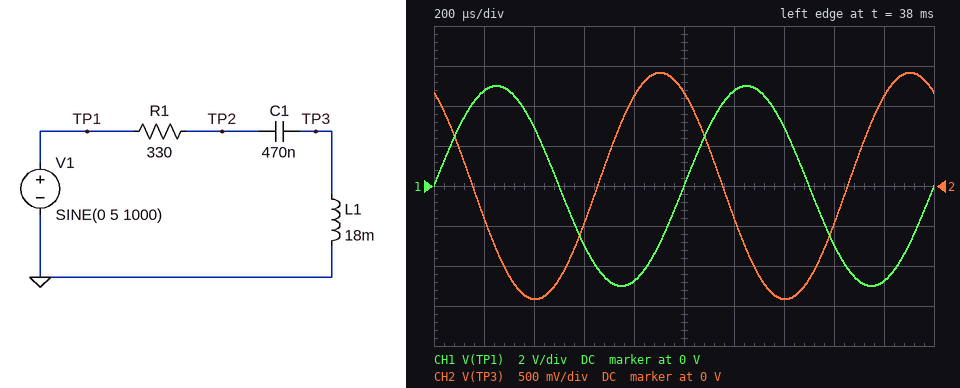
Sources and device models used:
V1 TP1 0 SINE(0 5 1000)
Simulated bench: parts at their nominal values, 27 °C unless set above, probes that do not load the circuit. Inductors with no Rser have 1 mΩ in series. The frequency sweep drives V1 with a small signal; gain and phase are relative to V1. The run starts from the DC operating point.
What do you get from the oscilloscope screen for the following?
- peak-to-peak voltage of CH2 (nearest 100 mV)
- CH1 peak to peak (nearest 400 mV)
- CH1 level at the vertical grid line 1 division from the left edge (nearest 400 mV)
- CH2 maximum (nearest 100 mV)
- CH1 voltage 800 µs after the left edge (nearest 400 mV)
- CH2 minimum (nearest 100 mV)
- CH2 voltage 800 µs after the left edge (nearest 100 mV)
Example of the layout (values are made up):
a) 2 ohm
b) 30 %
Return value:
a) 2.8 V
b) 10.0 V
c) 4.8 V
d) 1.4 V
e) -4.8 V
f) -1.4 V
g) 1.1 V
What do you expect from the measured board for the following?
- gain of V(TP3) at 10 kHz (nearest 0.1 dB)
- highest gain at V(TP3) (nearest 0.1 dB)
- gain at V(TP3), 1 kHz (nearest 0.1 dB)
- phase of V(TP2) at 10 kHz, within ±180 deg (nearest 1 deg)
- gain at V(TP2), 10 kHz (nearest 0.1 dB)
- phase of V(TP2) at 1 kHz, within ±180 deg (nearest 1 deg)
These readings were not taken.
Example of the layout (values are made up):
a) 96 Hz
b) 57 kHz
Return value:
a) -0.1 dB
b) 0 dB
c) -11.0 dB
d) 17 deg
e) -0.4 dB
f) -56 deg
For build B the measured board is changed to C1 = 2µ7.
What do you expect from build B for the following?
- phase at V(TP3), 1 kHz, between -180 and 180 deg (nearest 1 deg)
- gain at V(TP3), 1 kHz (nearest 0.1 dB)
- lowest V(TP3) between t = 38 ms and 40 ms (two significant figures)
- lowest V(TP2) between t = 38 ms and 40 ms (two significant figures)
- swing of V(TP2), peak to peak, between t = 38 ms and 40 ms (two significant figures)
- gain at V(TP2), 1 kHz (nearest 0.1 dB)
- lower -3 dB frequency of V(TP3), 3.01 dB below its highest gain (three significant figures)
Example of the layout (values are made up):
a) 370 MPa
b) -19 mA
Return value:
a) 81 deg
b) -9.4 dB
c) -1.7 V
d) -810 mV
e) 1.6 V
f) -15.8 dB
g) 2.74 kHz
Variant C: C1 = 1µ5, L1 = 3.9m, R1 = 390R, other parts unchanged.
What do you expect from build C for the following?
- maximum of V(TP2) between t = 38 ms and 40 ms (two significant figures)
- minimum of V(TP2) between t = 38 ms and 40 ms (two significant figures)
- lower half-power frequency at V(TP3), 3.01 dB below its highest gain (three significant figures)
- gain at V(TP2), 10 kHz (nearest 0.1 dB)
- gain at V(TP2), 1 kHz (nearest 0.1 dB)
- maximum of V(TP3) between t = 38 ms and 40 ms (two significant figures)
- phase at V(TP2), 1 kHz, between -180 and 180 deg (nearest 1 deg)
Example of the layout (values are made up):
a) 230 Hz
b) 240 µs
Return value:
a) 1.0 V
b) -1.0 V
c) 15.6 kHz
d) -5.8 dB
e) -13.8 dB
f) 310 mV
g) -78 deg
